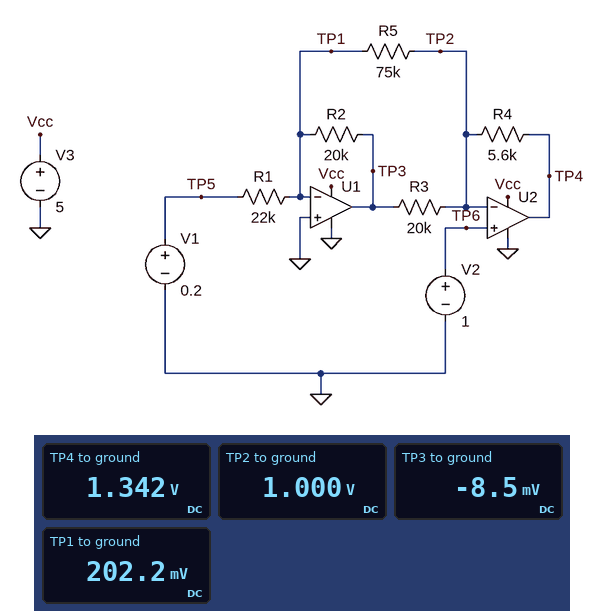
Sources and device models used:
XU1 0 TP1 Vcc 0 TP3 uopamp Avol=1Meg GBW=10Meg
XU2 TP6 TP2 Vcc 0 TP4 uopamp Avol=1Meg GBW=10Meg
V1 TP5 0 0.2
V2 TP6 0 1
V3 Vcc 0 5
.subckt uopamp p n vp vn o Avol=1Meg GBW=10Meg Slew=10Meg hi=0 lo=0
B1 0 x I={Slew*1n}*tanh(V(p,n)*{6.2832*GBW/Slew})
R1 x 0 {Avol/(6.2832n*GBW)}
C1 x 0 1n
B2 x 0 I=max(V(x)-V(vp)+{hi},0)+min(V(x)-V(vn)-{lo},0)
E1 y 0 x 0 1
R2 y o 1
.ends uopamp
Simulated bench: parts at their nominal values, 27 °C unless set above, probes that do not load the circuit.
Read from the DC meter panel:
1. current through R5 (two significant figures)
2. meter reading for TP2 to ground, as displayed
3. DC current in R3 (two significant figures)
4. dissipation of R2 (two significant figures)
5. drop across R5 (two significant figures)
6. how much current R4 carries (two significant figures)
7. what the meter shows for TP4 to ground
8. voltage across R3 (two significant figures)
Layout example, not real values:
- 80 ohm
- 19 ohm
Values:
- 11 µA
- 1.000 V
- 50 µA
- 2.2 µW
- 800 mV
- 61 µA
- 1.342 V
- 1.0 V
